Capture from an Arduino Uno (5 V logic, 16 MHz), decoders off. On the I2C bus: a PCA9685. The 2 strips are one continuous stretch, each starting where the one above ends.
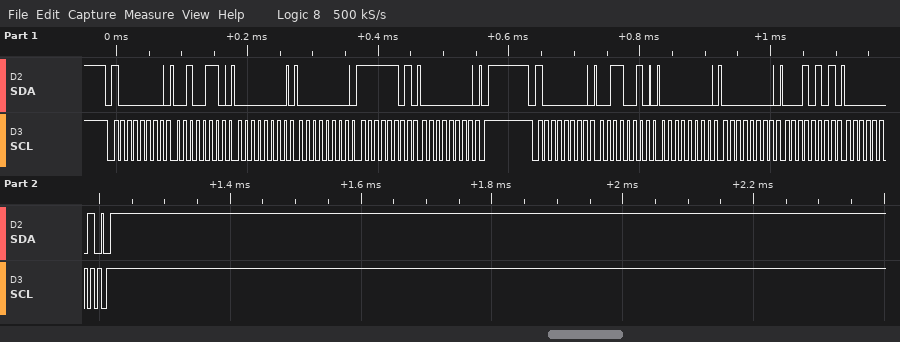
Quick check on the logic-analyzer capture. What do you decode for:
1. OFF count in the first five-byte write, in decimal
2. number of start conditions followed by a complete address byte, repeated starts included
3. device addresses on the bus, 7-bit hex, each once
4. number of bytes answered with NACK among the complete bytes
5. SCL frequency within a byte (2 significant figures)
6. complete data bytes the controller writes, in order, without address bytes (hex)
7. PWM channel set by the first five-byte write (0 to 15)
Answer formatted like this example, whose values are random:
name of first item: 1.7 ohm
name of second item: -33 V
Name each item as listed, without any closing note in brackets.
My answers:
OFF count in the first five-byte write, in decimal: 253
number of start conditions followed by a complete address byte, repeated starts included: 2
device addresses on the bus, 7-bit hex, each once: 0x40
number of bytes answered with NACK among the complete bytes: 0
SCL frequency within a byte: 100 kHz
complete data bytes the controller writes, in order, without address bytes: 26 00 00 FD 00 32 00 00 15 01
PWM channel set by the first five-byte write: 8
